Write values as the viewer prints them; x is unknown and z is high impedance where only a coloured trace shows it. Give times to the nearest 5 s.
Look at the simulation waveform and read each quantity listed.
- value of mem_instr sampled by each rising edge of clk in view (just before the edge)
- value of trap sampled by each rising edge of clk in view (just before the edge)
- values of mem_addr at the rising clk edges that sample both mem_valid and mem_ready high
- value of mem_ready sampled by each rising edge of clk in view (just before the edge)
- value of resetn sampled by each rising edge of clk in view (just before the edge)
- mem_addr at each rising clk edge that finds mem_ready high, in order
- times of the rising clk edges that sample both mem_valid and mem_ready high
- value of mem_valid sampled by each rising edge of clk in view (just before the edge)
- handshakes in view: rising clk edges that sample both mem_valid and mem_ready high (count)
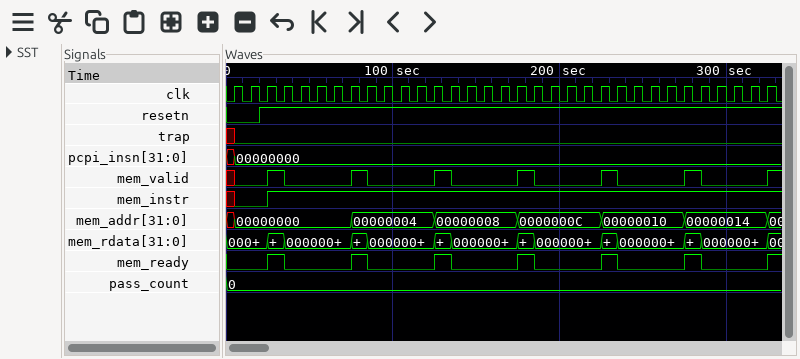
x 0 0 1 1 1 1 1 1 1 1 1 1 1 1 1 1 1 1 1 1 1 1 1 1 1 1 1 1 1 1 1 1
x 0 0 0 0 0 0 0 0 0 0 0 0 0 0 0 0 0 0 0 0 0 0 0 0 0 0 0 0 0 0 0 0
00000000, 00000004, 00000008, 0000000C, 00000010, 00000014
0 0 0 1 0 0 0 0 1 0 0 0 0 1 0 0 0 0 1 0 0 0 0 1 0 0 0 0 1 0 0 0 0
0 0 1 1 1 1 1 1 1 1 1 1 1 1 1 1 1 1 1 1 1 1 1 1 1 1 1 1 1 1 1 1 1
00000000, 00000004, 00000008, 0000000C, 00000010, 00000014
35 s, 85 s, 135 s, 185 s, 235 s, 285 s
x 0 0 1 0 0 0 0 1 0 0 0 0 1 0 0 0 0 1 0 0 0 0 1 0 0 0 0 1 0 0 0 0
6
